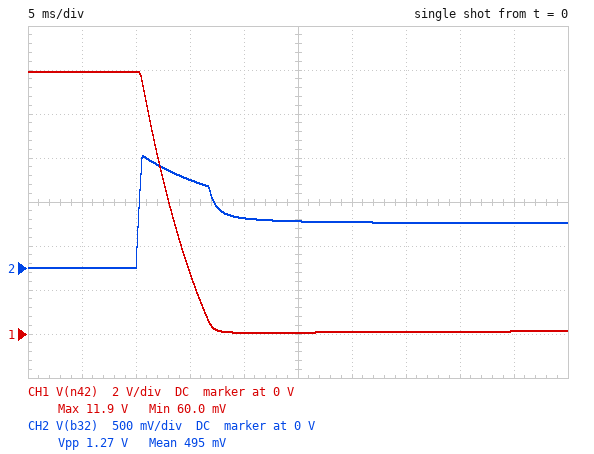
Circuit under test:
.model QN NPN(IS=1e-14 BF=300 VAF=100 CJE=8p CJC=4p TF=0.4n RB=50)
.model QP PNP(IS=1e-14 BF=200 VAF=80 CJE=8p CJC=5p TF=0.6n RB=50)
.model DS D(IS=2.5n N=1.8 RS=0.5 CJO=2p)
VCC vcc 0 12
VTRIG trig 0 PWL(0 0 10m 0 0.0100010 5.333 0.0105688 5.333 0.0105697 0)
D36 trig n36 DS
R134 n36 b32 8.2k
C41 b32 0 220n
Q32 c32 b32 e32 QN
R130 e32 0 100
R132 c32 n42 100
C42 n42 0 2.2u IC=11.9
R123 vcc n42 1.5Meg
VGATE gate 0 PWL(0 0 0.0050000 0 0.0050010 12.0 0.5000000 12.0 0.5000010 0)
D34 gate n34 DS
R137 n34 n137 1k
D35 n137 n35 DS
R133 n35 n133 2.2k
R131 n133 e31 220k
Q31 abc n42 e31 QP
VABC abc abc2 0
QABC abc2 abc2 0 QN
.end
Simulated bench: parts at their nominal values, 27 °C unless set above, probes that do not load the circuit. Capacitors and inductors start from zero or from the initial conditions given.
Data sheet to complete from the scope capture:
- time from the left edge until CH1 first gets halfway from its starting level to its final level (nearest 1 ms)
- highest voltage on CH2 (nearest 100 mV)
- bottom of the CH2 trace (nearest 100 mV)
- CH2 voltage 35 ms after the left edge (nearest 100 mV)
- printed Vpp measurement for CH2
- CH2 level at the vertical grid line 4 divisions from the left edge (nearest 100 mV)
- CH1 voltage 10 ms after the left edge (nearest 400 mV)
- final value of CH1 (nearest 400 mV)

13 ms
1.3 V
0 V
500 mV
1.27 V
600 mV
12.0 V
0 V
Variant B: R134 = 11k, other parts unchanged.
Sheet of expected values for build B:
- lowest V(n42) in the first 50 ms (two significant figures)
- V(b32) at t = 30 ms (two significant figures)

61 mV
660 mV
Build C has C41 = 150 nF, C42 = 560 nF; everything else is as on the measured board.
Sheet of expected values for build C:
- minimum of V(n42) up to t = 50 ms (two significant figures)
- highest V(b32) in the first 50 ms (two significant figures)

42 mV
1.7 V
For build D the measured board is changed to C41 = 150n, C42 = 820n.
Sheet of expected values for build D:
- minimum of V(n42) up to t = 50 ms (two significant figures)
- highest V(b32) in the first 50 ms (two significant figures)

47 mV
1.7 V
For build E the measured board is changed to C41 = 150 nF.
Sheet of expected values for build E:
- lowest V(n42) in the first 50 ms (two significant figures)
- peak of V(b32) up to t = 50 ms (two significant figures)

64 mV
1.7 V
